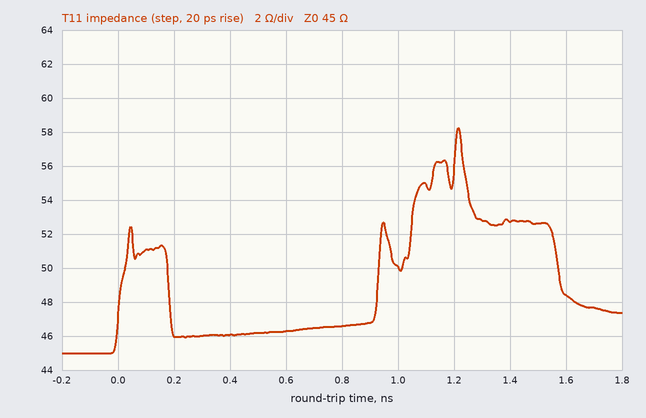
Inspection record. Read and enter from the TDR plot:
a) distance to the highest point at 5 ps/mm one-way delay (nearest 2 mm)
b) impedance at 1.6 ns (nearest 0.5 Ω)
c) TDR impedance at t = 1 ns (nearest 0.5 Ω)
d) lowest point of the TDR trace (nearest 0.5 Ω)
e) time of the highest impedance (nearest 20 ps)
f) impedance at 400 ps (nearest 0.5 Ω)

122 mm
48.5 Ω
50.0 Ω
45.0 Ω
1.22 ns
46.0 Ω
